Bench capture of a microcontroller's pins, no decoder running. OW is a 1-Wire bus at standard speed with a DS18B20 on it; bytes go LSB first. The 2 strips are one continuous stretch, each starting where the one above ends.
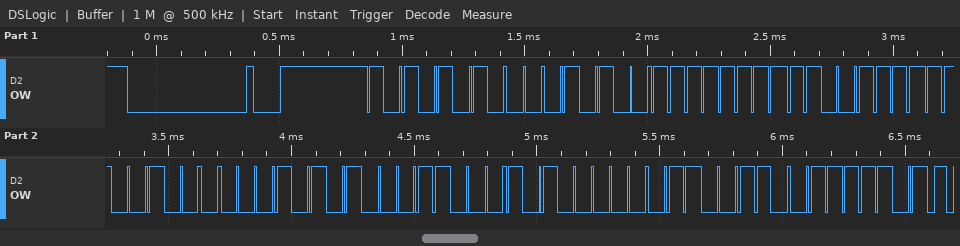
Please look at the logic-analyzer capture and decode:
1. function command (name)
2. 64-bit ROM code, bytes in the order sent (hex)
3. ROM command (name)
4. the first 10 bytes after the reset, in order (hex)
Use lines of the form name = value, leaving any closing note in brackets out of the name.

function command = Read Scratchpad
64-bit ROM code, bytes in the order sent = 28 FF F3 13 A8 18 05 66
ROM command = Match ROM
the first 10 bytes after the reset, in order = 55 28 FF F3 13 A8 18 05 66 BE
